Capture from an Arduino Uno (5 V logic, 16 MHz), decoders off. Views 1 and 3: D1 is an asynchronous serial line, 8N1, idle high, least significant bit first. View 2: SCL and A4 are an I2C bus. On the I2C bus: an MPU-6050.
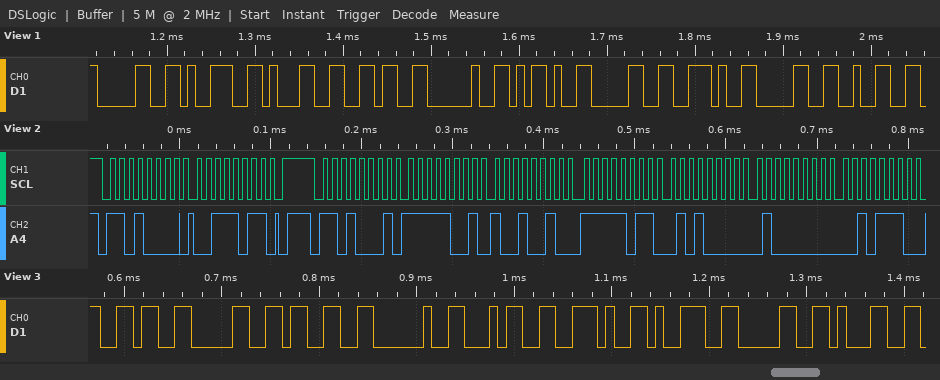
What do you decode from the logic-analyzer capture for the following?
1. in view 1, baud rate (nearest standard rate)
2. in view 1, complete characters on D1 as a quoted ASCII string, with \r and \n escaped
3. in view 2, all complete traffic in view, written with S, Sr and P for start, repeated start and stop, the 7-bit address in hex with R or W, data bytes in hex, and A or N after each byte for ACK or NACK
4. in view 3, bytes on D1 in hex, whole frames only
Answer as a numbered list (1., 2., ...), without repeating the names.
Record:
1. 115200 baud
2. "0916 -0.02"
3. S 68W A 3B A P S 68R A F9 A 92 A FB A 50 A 40 A 2E A
4. 36 30 33 20 34 2E 39 30 31
